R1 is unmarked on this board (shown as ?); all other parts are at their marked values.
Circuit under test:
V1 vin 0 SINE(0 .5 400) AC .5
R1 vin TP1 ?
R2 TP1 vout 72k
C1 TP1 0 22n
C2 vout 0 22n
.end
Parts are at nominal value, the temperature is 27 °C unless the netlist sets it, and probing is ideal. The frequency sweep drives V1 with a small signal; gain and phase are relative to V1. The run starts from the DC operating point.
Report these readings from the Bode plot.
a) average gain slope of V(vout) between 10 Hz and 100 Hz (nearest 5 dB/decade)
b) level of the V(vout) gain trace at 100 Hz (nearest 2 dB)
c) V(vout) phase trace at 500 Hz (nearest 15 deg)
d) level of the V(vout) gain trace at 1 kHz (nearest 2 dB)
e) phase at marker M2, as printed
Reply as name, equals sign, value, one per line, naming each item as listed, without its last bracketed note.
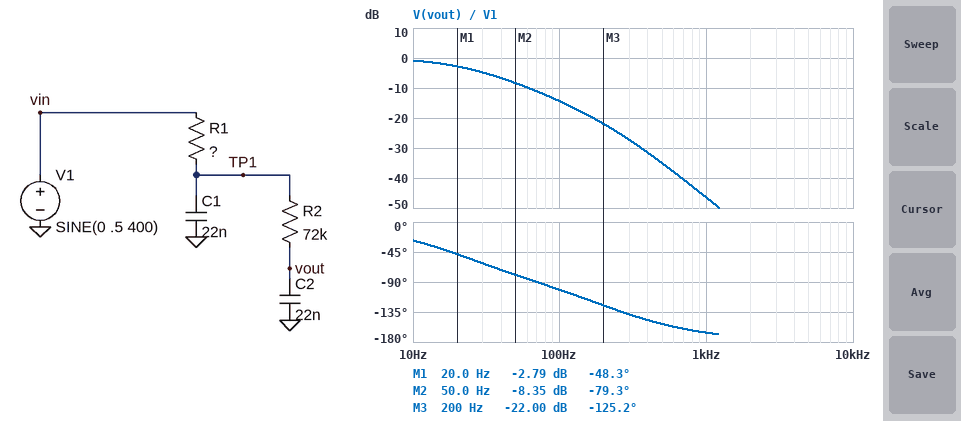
average gain slope of V(vout) between 10 Hz and 100 Hz = -15 dB/decade
level of the V(vout) gain trace at 100 Hz = -14 dB
V(vout) phase trace at 500 Hz = -150 deg
level of the V(vout) gain trace at 1 kHz = -46 dB
phase at marker M2, as printed = -79.3 deg
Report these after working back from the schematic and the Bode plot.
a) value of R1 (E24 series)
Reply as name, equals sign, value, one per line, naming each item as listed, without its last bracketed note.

value of R1 = 150 kΩ
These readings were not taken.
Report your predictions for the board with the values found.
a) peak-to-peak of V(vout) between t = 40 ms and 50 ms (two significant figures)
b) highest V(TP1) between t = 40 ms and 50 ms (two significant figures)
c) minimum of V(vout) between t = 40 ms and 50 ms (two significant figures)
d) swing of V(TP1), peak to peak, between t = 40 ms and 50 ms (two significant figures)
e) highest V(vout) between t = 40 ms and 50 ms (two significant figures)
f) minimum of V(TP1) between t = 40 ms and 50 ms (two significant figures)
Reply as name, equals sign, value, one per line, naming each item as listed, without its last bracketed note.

peak-to-peak of V(vout) between t = 40 ms and 50 ms = 26 mV
highest V(TP1) between t = 40 ms and 50 ms = 54 mV
minimum of V(vout) between t = 40 ms and 50 ms = -13 mV
swing of V(TP1), peak to peak, between t = 40 ms and 50 ms = 110 mV
highest V(vout) between t = 40 ms and 50 ms = 13 mV
minimum of V(TP1) between t = 40 ms and 50 ms = -54 mV
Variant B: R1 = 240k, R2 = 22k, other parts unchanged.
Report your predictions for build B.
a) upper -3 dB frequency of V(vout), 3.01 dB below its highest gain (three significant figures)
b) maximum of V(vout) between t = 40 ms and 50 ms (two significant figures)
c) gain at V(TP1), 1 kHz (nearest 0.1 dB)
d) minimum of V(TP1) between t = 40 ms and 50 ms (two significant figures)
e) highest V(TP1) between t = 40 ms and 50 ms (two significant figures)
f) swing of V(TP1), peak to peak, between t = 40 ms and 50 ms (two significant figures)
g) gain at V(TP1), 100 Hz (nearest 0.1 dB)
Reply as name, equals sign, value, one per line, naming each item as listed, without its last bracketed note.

upper -3 dB frequency of V(vout), 3.01 dB below its highest gain = 14.7 Hz
maximum of V(vout) between t = 40 ms and 50 ms = 16 mV
gain at V(TP1), 1 kHz = -31.6 dB
minimum of V(TP1) between t = 40 ms and 50 ms = -25 mV
highest V(TP1) between t = 40 ms and 50 ms = 25 mV
swing of V(TP1), peak to peak, between t = 40 ms and 50 ms = 50 mV
gain at V(TP1), 100 Hz = -16.4 dB
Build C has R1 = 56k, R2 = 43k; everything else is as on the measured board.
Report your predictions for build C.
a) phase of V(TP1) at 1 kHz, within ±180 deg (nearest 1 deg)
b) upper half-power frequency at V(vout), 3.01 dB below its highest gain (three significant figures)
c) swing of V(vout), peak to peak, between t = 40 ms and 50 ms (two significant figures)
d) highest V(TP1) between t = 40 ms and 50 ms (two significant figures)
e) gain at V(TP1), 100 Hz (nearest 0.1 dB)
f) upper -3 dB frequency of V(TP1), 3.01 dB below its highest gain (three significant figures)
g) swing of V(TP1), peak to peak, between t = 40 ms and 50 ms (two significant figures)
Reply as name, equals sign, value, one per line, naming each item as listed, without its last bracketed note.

phase of V(TP1) at 1 kHz, within ±180 deg = -74 deg
upper half-power frequency at V(vout), 3.01 dB below its highest gain = 51.8 Hz
swing of V(vout), peak to peak, between t = 40 ms and 50 ms = 94 mV
highest V(TP1) between t = 40 ms and 50 ms = 120 mV
gain at V(TP1), 100 Hz = -5.6 dB
upper -3 dB frequency of V(TP1), 3.01 dB below its highest gain = 57.4 Hz
swing of V(TP1), peak to peak, between t = 40 ms and 50 ms = 240 mV
